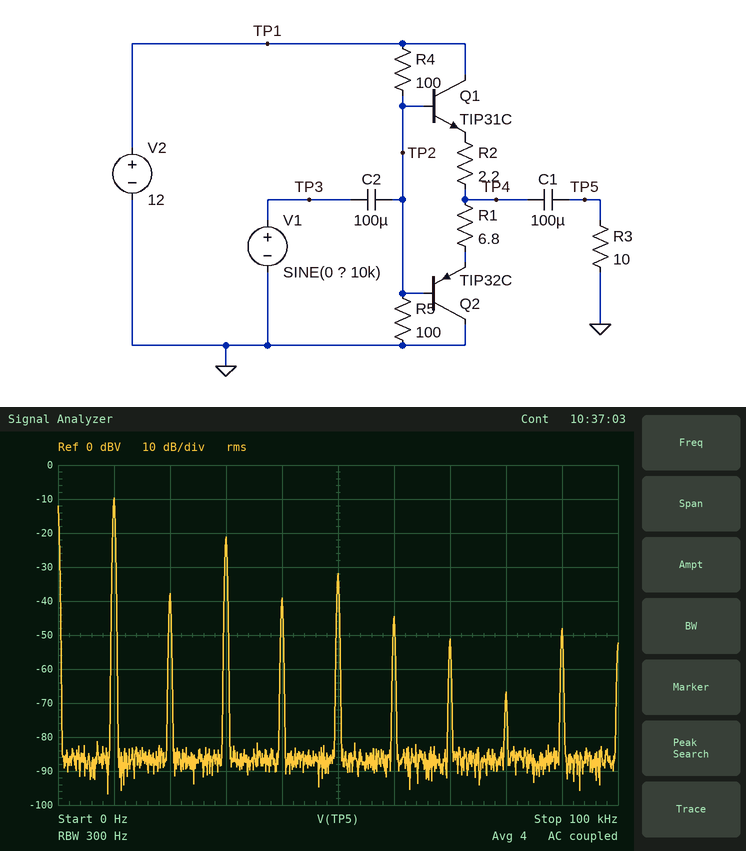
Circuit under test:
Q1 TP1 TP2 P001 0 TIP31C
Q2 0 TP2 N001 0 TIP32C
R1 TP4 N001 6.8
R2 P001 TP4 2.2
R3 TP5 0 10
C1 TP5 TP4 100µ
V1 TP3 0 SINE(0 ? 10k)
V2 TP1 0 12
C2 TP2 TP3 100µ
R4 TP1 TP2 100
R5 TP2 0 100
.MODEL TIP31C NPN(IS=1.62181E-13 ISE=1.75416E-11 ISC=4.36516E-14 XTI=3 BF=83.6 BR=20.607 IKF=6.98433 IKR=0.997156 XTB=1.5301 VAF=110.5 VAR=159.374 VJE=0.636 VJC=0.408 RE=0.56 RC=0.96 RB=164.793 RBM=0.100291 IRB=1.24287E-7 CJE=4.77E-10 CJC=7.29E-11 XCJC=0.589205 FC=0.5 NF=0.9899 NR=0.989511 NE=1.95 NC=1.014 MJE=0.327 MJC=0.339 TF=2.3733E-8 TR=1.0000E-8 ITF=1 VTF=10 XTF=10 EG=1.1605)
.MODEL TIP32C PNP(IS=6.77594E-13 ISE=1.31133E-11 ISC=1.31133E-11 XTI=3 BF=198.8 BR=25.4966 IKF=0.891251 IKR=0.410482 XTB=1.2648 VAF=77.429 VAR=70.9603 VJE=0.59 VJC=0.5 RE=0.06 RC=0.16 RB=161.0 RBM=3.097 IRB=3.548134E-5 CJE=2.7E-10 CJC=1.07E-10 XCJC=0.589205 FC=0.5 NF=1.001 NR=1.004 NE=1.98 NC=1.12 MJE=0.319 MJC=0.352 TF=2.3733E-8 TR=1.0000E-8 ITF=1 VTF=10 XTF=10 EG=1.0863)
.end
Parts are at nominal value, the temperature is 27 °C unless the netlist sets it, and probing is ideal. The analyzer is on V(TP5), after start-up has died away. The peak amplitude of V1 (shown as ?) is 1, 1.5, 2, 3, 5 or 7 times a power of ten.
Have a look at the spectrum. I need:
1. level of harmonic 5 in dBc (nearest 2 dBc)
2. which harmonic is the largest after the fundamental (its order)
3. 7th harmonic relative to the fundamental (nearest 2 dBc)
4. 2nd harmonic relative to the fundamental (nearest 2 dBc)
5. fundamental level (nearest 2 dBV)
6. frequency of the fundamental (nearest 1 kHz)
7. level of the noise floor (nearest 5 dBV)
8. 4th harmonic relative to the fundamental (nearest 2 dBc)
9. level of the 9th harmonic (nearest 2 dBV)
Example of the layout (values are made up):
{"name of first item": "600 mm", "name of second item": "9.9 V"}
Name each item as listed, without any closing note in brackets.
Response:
{"level of harmonic 5 in dBc": "-22 dBc", "which harmonic is the largest after the fundamental": "3", "7th harmonic relative to the fundamental": "-42 dBc", "2nd harmonic relative to the fundamental": "-28 dBc", "fundamental level": "-10 dBV", "frequency of the fundamental": "10 kHz", "level of the noise floor": "-85 dBV", "4th harmonic relative to the fundamental": "-30 dBc", "level of the 9th harmonic": "-48 dBV"}
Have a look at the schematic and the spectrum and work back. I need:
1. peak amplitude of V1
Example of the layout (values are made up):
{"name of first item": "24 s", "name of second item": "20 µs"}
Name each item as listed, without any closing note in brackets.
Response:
{"peak amplitude of V1": "1.5 V"}
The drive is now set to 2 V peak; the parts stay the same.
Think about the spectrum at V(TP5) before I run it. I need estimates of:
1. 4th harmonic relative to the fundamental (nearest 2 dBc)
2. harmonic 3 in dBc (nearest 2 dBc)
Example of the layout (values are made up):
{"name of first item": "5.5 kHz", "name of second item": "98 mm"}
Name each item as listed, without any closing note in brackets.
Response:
{"4th harmonic relative to the fundamental": "-32 dBc", "harmonic 3 in dBc": "-14 dBc"}
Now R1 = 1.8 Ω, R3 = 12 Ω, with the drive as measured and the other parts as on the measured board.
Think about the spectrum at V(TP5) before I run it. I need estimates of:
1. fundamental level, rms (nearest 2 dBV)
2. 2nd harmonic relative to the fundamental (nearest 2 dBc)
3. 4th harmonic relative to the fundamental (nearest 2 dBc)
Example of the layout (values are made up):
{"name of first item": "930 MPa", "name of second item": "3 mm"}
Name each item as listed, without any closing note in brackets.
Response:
{"fundamental level, rms": "-8 dBV", "2nd harmonic relative to the fundamental": "-42 dBc", "4th harmonic relative to the fundamental": "-44 dBc"}
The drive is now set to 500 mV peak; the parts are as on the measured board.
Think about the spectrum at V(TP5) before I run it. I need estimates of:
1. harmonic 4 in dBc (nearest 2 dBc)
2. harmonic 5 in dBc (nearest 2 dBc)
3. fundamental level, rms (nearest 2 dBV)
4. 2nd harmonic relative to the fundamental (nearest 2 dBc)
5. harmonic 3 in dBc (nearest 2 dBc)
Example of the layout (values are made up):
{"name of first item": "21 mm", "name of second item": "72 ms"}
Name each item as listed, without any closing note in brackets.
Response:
{"harmonic 4 in dBc": "-12 dBc", "harmonic 5 in dBc": "-8 dBc", "fundamental level, rms": "-70 dBV", "2nd harmonic relative to the fundamental": "-10 dBc", "harmonic 3 in dBc": "-4 dBc"}
